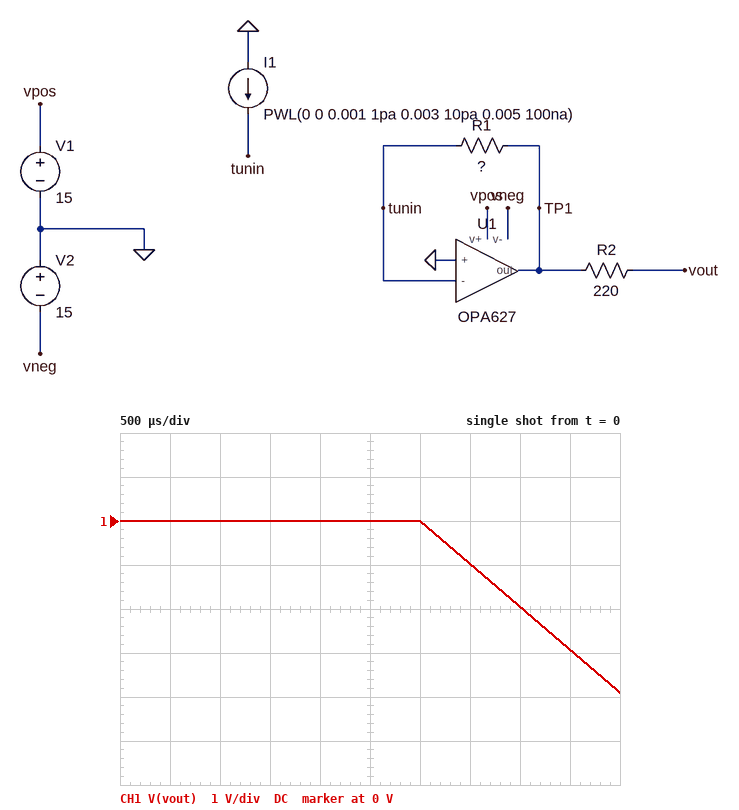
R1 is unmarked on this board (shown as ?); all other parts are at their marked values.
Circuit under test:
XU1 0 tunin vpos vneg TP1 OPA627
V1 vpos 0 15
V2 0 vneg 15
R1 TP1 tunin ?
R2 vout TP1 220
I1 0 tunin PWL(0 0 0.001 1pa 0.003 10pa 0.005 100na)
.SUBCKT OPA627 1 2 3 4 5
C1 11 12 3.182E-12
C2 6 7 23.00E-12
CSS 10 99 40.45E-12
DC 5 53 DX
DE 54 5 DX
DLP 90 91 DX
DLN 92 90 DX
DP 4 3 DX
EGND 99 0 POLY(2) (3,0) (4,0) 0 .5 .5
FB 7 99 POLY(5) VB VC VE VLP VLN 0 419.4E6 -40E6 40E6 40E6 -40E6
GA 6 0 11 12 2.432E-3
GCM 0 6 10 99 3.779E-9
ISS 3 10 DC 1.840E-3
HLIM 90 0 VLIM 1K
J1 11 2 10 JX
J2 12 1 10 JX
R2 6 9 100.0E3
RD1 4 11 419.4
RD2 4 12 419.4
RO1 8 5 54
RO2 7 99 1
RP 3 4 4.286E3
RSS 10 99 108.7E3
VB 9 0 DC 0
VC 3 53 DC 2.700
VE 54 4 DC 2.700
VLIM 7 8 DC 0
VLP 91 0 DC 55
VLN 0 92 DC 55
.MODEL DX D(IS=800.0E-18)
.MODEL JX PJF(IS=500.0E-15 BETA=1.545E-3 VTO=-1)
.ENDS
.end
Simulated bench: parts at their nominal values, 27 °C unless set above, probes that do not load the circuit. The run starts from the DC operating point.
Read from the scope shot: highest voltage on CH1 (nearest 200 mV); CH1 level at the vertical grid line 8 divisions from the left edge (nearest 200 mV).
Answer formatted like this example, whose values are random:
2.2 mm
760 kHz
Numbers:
0 V
-2.0 V
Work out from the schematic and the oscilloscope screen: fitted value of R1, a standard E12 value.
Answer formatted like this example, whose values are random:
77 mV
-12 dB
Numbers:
39 MΩ
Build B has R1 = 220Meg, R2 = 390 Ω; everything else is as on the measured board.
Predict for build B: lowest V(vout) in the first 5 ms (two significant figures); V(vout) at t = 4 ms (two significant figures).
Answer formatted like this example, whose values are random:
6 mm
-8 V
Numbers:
-13 V
-11 V
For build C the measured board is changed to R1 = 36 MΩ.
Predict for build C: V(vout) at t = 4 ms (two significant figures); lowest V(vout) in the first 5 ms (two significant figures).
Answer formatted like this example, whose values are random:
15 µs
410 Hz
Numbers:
-1.8 V
-3.6 V
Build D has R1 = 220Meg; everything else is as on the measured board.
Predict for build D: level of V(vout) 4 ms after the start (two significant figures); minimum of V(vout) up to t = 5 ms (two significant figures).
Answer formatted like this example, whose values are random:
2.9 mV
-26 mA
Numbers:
-11 V
-13 V
